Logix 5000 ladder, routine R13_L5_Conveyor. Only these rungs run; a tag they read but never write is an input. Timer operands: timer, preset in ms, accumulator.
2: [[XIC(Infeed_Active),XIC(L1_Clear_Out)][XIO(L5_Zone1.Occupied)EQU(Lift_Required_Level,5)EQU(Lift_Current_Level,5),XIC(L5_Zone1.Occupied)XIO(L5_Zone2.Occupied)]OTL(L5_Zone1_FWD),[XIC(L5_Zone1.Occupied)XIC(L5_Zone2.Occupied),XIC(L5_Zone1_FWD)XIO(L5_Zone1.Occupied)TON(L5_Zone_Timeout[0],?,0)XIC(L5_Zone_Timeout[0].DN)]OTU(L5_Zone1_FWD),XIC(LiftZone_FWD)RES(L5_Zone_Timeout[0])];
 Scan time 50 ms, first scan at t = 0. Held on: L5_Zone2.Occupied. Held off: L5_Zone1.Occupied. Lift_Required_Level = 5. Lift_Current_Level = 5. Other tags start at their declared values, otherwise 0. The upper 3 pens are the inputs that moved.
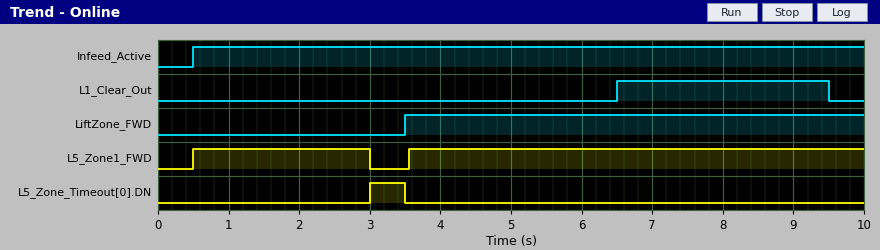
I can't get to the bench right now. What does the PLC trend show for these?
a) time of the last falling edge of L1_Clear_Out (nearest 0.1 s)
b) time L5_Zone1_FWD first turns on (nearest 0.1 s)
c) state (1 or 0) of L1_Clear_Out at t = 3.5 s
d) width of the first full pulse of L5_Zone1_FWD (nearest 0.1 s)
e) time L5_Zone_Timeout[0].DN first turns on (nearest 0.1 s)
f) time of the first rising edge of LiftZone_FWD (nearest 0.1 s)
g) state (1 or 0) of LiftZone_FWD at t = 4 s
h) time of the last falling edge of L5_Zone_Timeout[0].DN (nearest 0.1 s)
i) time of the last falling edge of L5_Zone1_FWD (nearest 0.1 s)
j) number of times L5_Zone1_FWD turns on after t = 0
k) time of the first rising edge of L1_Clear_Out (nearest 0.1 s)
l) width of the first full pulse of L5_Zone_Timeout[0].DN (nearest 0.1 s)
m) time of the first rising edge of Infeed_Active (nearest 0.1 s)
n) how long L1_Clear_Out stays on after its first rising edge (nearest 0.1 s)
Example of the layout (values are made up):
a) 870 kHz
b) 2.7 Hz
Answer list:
a) 9.5 s
b) 0.5 s
c) 0
d) 2.5 s
e) 3.0 s
f) 3.5 s
g) 1
h) 3.5 s
i) 3.0 s
j) 2
k) 6.5 s
l) 0.5 s
m) 0.5 s
n) 3.0 s
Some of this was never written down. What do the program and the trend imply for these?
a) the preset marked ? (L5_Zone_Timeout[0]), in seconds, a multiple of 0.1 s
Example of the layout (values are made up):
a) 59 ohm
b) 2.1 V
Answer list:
a) 2.5 s
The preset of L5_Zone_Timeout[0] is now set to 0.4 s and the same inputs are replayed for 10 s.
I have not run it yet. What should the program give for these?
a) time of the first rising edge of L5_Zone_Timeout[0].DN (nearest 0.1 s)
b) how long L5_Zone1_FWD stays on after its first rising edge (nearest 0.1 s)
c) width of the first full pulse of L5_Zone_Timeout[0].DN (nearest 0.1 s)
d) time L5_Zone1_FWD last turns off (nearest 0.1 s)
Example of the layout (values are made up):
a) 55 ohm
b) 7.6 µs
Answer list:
a) 0.9 s
b) 0.4 s
c) 2.6 s
d) 0.9 s
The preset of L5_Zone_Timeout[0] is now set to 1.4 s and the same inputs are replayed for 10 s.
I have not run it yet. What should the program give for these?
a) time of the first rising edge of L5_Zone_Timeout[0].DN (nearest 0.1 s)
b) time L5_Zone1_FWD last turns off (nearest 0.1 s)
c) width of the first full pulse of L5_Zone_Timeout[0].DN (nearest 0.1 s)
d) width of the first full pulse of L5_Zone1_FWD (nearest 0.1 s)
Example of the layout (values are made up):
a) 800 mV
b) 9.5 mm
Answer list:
a) 1.9 s
b) 1.9 s
c) 1.6 s
d) 1.4 s
